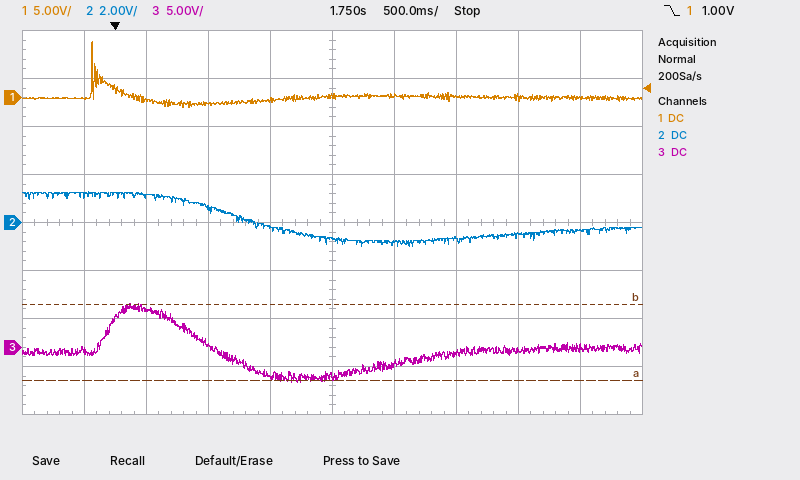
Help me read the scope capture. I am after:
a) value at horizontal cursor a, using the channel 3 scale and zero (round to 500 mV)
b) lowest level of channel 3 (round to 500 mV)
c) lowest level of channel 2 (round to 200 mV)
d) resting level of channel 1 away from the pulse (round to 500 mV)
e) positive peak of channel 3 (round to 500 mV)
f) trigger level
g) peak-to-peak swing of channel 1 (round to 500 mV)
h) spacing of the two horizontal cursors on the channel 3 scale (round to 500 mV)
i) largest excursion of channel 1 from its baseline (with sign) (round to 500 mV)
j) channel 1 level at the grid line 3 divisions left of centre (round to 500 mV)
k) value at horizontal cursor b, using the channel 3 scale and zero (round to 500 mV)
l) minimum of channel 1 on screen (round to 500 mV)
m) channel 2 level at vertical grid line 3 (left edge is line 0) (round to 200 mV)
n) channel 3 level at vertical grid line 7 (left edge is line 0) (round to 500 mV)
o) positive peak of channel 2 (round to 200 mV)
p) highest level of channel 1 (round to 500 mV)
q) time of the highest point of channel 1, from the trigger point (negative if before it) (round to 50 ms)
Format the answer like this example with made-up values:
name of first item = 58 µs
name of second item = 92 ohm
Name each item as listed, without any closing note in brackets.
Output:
value at horizontal cursor a, using the channel 3 scale and zero = -3.5 V
lowest level of channel 3 = -3.5 V
lowest level of channel 2 = -1.0 V
resting level of channel 1 away from the pulse = 0.0 V
positive peak of channel 3 = 4.5 V
trigger level = 1.00 V
peak-to-peak swing of channel 1 = 7.0 V
spacing of the two horizontal cursors on the channel 3 scale = 8.0 V
largest excursion of channel 1 from its baseline (with sign) = +6.0 V
channel 1 level at the grid line 3 divisions left of centre = 0.0 V
value at horizontal cursor b, using the channel 3 scale and zero = 4.5 V
minimum of channel 1 on screen = -1.0 V
channel 2 level at vertical grid line 3 (left edge is line 0) = 600 mV
channel 3 level at vertical grid line 7 (left edge is line 0) = -500 mV
positive peak of channel 2 = 1.2 V
highest level of channel 1 = 6.0 V
time of the highest point of channel 1, from the trigger point (negative if before it) = -200 ms
